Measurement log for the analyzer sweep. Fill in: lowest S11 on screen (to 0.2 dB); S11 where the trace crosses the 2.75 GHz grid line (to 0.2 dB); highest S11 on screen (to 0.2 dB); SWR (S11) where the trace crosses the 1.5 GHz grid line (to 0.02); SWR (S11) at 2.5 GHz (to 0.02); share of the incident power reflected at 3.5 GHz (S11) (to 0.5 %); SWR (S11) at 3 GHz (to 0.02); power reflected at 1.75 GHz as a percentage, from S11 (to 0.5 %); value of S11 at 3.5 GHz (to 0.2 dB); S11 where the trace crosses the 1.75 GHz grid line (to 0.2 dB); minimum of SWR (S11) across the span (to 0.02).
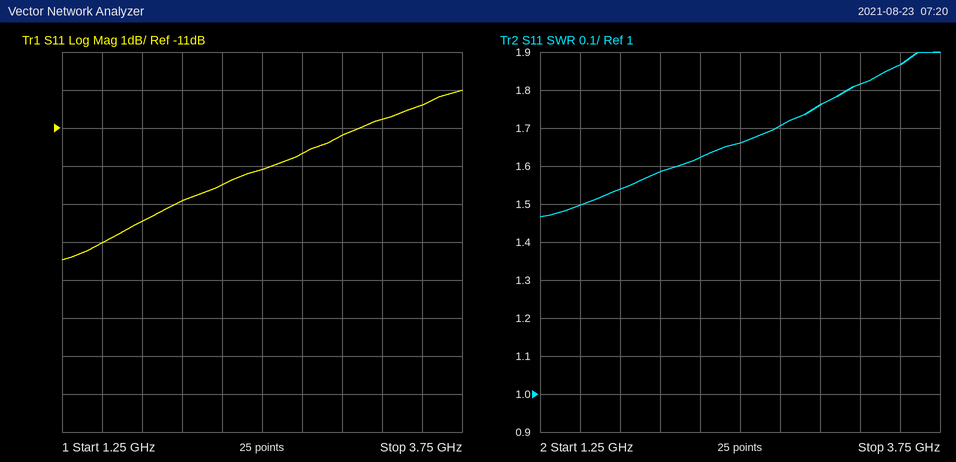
-14.4 dB
-11.6 dB
-10.0 dB
1.50
1.66
9.0 %
1.76
4.5 %
-10.4 dB
-13.4 dB
1.46
